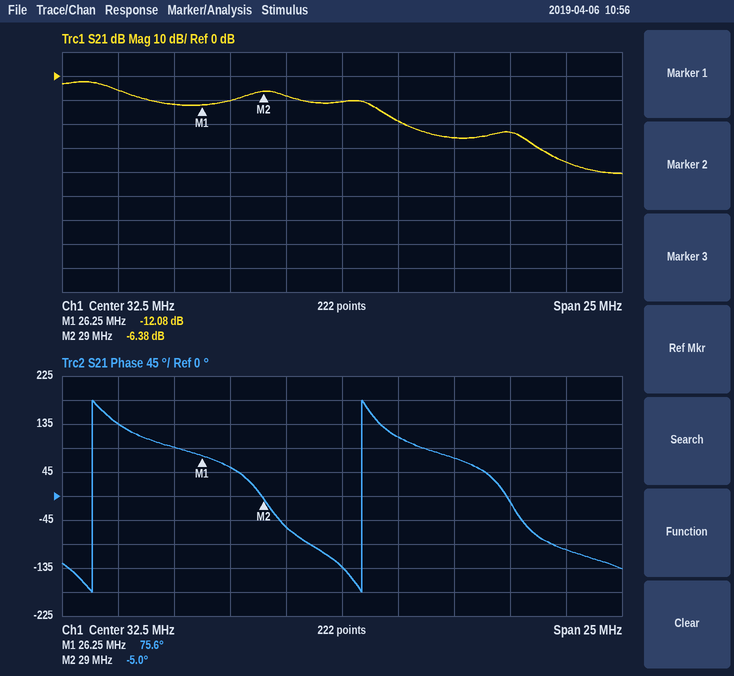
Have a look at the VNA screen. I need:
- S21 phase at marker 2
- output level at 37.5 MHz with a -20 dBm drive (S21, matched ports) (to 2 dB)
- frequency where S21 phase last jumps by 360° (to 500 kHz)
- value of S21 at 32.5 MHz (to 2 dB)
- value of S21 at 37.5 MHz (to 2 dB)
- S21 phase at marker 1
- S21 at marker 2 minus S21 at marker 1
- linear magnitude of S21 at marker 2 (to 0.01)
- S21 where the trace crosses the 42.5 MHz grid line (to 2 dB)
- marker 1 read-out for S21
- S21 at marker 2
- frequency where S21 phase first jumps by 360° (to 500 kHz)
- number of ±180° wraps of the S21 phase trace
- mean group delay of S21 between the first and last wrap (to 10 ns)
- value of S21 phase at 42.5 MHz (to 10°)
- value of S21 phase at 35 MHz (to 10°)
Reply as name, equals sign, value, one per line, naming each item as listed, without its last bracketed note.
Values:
S21 phase at marker 2 = -5.0°
output level at 37.5 MHz with a -20 dBm drive (S21, matched ports) = -46 dBm
frequency where S21 phase last jumps by 360° = 33.5 MHz
value of S21 at 32.5 MHz = -10 dB
value of S21 at 37.5 MHz = -26 dB
S21 phase at marker 1 = 75.6°
S21 at marker 2 minus S21 at marker 1 = 5.70 dB
linear magnitude of S21 at marker 2 = 0.48
S21 where the trace crosses the 42.5 MHz grid line = -36 dB
marker 1 read-out for S21 = -12.08 dB
S21 at marker 2 = -6.38 dB
frequency where S21 phase first jumps by 360° = 21.5 MHz
number of ±180° wraps of the S21 phase trace = 2
mean group delay of S21 between the first and last wrap = 80 ns
value of S21 phase at 42.5 MHz = -100°
value of S21 phase at 35 MHz = 110°
